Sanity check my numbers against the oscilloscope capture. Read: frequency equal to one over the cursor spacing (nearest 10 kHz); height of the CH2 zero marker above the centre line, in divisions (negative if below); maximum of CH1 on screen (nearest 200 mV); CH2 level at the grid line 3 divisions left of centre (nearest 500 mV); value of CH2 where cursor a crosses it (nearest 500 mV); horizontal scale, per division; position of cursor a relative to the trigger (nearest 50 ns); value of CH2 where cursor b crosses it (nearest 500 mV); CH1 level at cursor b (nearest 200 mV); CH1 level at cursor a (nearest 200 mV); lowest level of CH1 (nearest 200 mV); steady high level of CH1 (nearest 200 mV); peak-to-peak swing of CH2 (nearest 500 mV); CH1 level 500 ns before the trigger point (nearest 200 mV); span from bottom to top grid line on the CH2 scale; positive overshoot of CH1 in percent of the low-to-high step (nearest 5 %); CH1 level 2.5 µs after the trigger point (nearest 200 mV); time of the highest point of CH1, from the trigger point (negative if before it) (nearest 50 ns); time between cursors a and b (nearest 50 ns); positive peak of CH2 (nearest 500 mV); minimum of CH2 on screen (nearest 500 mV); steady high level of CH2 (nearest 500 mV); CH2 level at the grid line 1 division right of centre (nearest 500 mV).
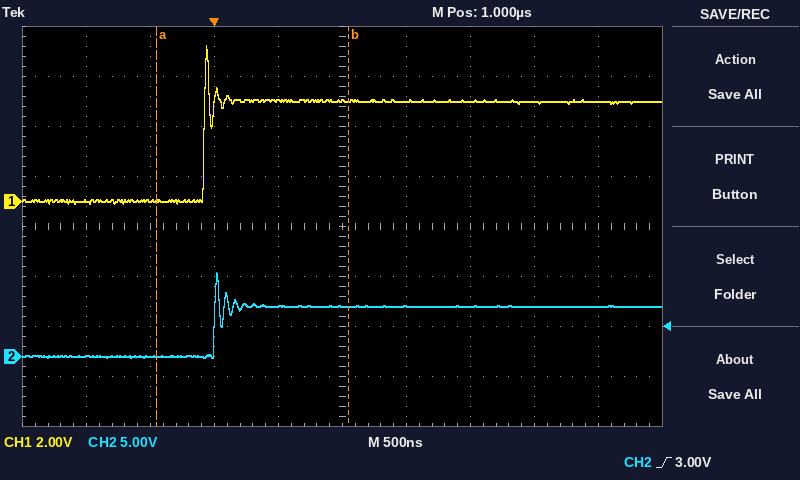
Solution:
670 kHz
-2.6 div
6.2 V
0.0 V
0.0 V
500 ns
-450 ns
5.0 V
4.0 V
0.0 V
0.0 V
4.0 V
8.5 V
0.0 V
40 V
55 %
4.0 V
-50 ns
1.50 µs
8.5 V
0.0 V
5.0 V
5.0 V
